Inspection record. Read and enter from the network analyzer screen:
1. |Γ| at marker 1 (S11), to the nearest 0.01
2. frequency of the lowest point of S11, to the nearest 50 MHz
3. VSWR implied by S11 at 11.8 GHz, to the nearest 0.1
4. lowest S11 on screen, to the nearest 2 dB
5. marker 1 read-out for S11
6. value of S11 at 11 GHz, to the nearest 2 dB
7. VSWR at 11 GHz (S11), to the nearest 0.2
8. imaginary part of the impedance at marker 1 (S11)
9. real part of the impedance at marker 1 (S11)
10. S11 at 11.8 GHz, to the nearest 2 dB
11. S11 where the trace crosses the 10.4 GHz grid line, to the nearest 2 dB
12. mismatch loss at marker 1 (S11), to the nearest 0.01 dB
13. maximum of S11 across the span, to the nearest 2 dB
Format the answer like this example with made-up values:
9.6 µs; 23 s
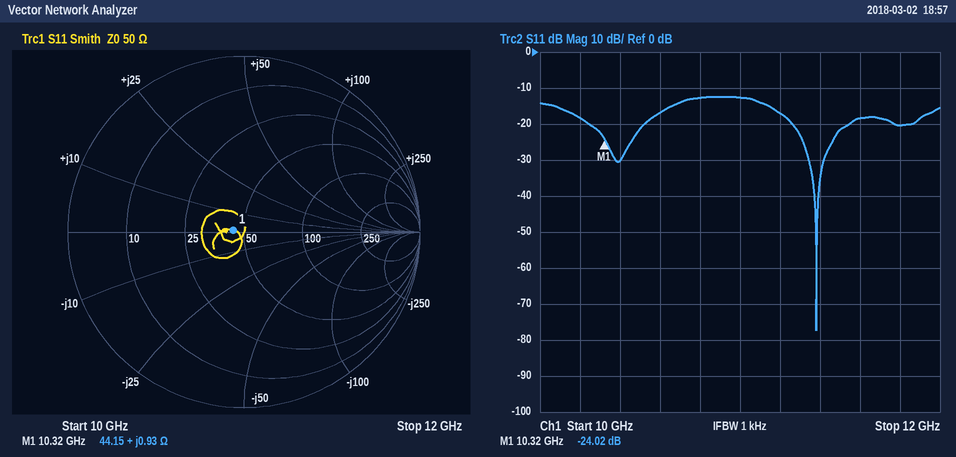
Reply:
0.06; 11.40 GHz; 1.2; -78 dB; -24.02 dB; -12 dB; 1.6; +0.93 Ω; 44.15 Ω; -20 dB; -30 dB; 0.02 dB; -12 dB
